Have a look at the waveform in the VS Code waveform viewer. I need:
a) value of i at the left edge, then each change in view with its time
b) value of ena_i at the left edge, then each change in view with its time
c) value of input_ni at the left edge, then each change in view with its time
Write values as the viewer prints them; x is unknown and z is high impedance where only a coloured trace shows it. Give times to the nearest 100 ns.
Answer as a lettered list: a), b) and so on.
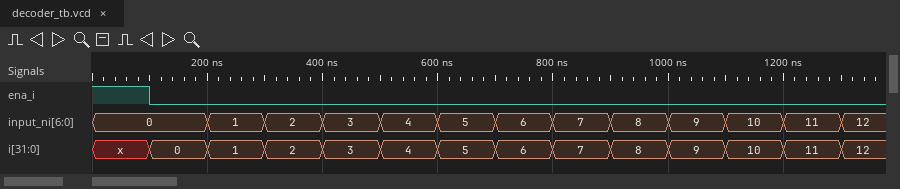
a) x, 0 at 100 ns, 1 at 200 ns, 2 at 300 ns, 3 at 400 ns, 4 at 500 ns, 5 at 600 ns, 6 at 700 ns, 7 at 800 ns, 8 at 900 ns, 9 at 1000 ns, 10 at 1100 ns, 11 at 1200 ns, 12 at 1300 ns
b) 1, 0 at 100 ns
c) 0, 1 at 200 ns, 2 at 300 ns, 3 at 400 ns, 4 at 500 ns, 5 at 600 ns, 6 at 700 ns, 7 at 800 ns, 8 at 900 ns, 9 at 1000 ns, 10 at 1100 ns, 11 at 1200 ns, 12 at 1300 ns
